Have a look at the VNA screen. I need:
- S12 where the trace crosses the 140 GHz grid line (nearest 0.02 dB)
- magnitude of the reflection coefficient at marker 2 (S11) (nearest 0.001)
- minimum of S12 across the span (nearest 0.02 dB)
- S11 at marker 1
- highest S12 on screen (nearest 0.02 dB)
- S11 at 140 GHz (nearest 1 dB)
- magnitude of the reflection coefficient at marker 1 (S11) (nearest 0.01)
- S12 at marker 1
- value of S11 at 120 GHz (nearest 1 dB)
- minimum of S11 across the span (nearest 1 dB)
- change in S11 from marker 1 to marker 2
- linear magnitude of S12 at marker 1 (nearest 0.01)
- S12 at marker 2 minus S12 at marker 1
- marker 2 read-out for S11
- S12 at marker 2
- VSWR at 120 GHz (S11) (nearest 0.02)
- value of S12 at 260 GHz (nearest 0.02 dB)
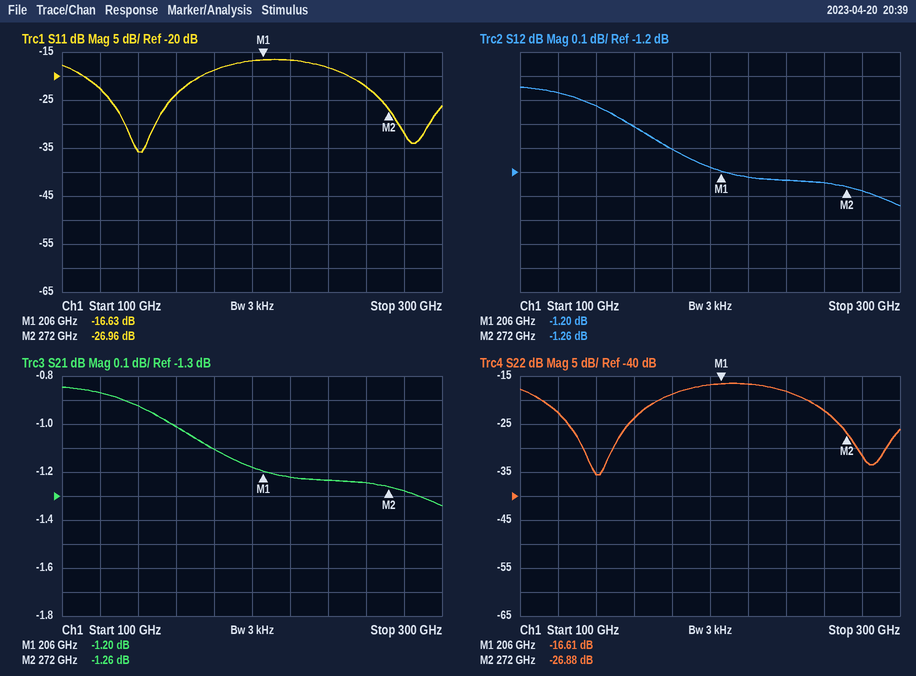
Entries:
-0.92 dB
0.045
-1.34 dB
-16.63 dB
-0.84 dB
-36 dB
0.15
-1.20 dB
-23 dB
-36 dB
-10.33 dB
0.87
-0.06 dB
-26.96 dB
-1.26 dB
1.16
-1.24 dB
